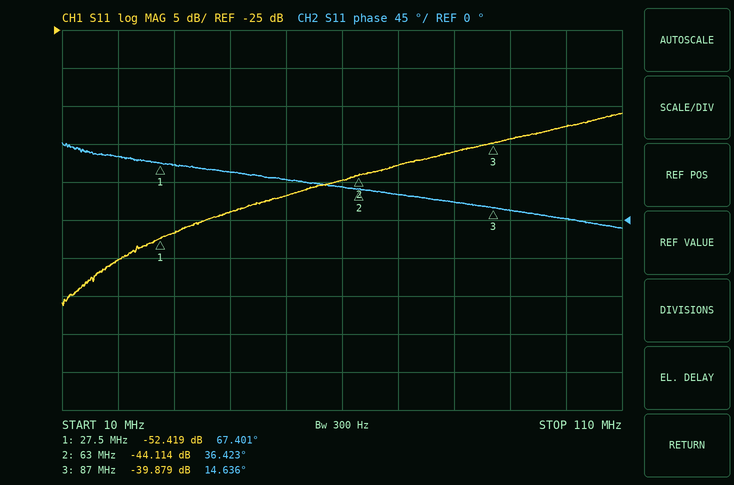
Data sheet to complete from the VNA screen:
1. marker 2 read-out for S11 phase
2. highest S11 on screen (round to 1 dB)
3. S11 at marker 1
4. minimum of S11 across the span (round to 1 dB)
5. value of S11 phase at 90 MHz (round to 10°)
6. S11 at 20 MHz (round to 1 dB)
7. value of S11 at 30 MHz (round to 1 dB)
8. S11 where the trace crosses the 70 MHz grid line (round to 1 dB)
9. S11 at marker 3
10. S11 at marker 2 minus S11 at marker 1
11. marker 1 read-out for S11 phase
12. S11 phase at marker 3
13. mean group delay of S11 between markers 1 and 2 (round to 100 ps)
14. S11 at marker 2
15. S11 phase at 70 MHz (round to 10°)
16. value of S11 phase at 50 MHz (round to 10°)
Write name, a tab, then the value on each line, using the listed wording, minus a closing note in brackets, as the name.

marker 2 read-out for S11 phase	36.423°
highest S11 on screen	-36 dB
S11 at marker 1	-52.419 dB
minimum of S11 across the span	-61 dB
value of S11 phase at 90 MHz	10°
S11 at 20 MHz	-55 dB
value of S11 at 30 MHz	-52 dB
S11 where the trace crosses the 70 MHz grid line	-43 dB
S11 at marker 3	-39.879 dB
S11 at marker 2 minus S11 at marker 1	8.305 dB
marker 1 read-out for S11 phase	67.401°
S11 phase at marker 3	14.636°
mean group delay of S11 between markers 1 and 2	2.4 ns
S11 at marker 2	-44.114 dB
S11 phase at 70 MHz	30°
value of S11 phase at 50 MHz	50°
